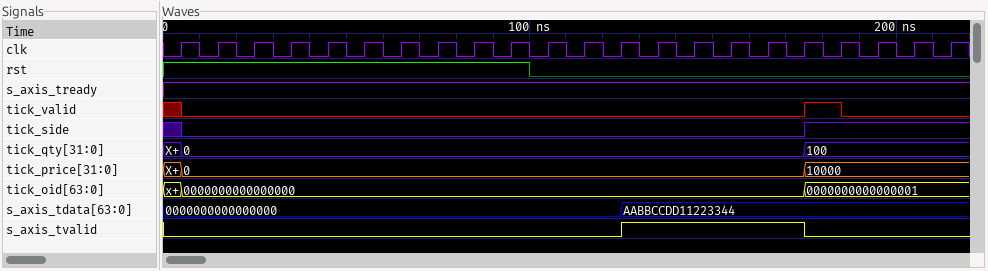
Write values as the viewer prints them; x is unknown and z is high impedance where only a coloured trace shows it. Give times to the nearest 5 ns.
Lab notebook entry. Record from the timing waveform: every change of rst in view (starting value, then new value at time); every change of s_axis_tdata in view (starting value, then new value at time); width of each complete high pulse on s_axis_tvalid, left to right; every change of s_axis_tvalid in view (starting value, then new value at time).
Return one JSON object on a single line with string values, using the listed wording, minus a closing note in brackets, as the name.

{"every change of rst in view": "1, 0 at 100 ns", "every change of s_axis_tdata in view": "0000000000000000, AABBCCDD11223344 at 125 ns", "width of each complete high pulse on s_axis_tvalid, left to right": "50 ns", "every change of s_axis_tvalid in view": "0, 1 at 125 ns, 0 at 175 ns"}
